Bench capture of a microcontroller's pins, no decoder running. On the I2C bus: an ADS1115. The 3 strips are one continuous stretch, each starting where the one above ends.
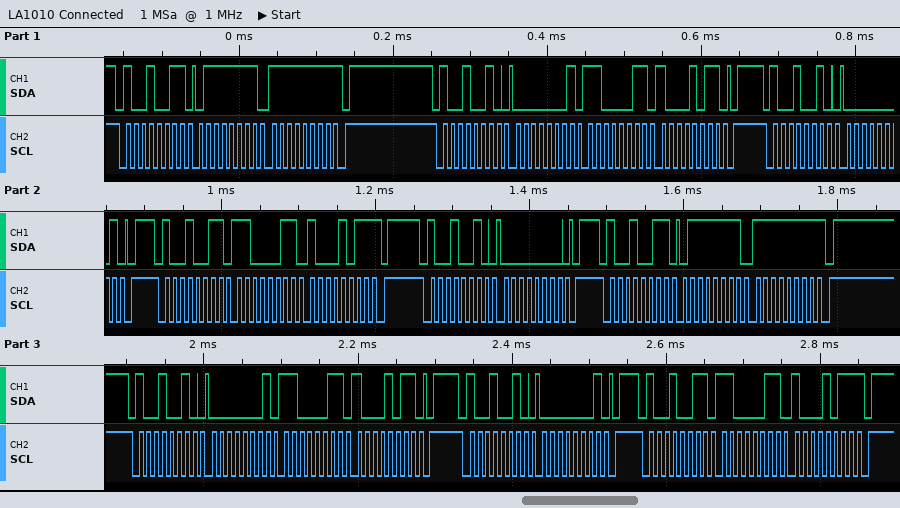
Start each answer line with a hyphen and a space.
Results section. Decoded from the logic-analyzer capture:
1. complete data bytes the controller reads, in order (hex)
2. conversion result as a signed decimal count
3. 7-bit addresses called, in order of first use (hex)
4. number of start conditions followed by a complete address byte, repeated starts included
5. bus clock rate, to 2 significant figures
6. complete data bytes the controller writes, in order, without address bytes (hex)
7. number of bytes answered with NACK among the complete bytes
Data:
- 7F FF C3 8B 7F FF C3 8B
- 32767
- 0x49
- 9
- 100 kHz
- 01 C3 8B 01 00 01 C3 8B 01
- 4
